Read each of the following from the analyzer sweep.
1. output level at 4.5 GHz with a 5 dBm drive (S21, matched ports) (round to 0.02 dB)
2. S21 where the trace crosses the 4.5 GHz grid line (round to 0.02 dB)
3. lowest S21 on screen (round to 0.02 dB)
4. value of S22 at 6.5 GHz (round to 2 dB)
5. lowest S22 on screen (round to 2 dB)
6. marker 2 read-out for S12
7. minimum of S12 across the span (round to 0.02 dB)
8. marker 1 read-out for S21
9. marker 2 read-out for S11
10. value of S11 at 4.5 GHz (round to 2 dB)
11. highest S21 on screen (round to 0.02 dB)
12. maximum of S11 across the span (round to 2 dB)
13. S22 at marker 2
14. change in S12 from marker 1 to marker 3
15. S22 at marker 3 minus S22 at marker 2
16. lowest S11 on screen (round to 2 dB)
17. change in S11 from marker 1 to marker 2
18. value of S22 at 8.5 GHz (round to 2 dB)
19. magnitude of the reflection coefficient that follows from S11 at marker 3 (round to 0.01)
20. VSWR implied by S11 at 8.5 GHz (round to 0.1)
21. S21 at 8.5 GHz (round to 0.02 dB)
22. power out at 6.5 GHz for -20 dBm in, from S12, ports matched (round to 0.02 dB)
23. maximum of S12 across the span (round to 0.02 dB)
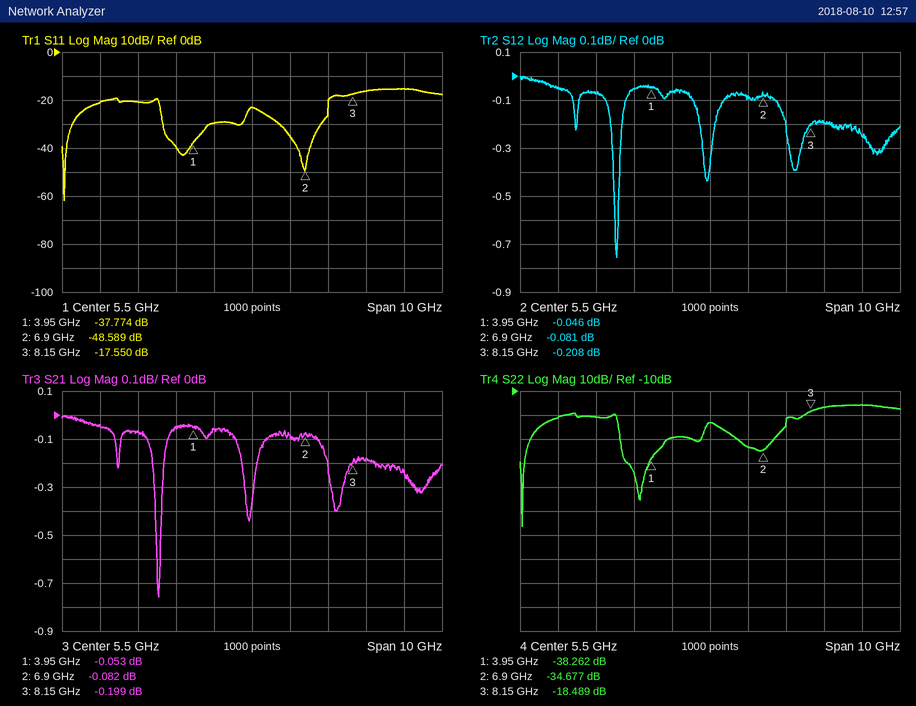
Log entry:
4.94 dBm
-0.06 dB
-0.76 dB
-34 dB
-66 dB
-0.081 dB
-0.76 dB
-0.053 dB
-48.589 dB
-30 dB
0.00 dB
-16 dB
-34.677 dB
-0.162 dB
16.188 dB
-62 dB
-10.815 dB
-16 dB
0.13
1.4
-0.18 dB
-20.08 dBm
0.00 dB
